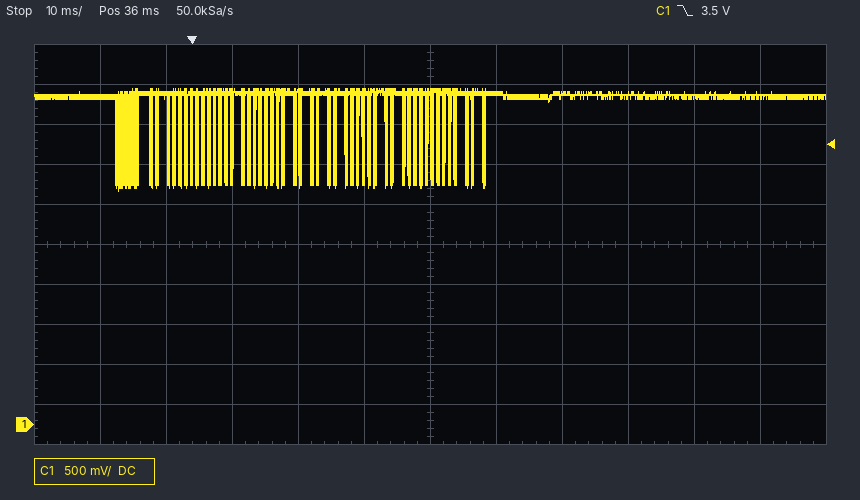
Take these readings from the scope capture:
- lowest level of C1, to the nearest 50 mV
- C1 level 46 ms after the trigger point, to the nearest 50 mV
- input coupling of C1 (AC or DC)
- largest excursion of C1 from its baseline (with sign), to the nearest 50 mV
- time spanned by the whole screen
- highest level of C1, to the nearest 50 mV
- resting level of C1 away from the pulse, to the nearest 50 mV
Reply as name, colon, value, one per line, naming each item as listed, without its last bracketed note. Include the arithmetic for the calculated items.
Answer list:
lowest level of C1, to the nearest 50 mV: 2.90 V
C1 level 46 ms after the trigger point, to the nearest 50 mV: 4.15 V
input coupling of C1: DC
largest excursion of C1 from its baseline (with sign), to the nearest 50 mV: 2.90 V − (4.10 V) = -1.20 V
time spanned by the whole screen: 120 ms
highest level of C1, to the nearest 50 mV: 4.20 V
resting level of C1 away from the pulse, to the nearest 50 mV: 4.10 V
